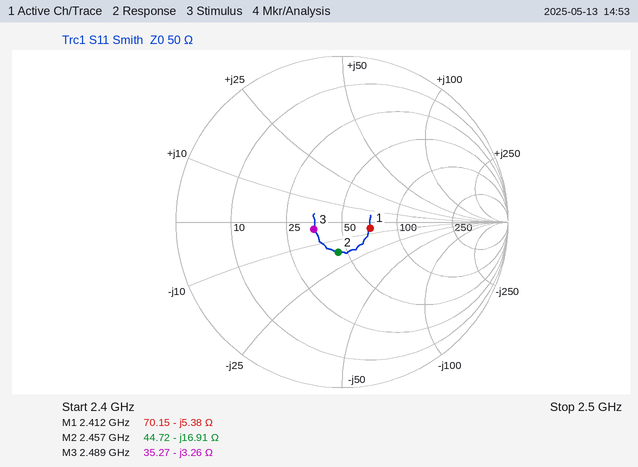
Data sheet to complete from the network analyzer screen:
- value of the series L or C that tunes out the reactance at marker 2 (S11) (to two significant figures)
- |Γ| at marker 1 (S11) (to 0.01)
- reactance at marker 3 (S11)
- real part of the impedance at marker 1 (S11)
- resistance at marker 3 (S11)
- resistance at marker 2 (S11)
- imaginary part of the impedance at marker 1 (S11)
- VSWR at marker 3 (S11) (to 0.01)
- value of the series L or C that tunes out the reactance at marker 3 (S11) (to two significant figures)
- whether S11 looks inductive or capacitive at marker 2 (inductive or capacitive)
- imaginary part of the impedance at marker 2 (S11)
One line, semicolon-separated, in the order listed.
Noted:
1.1 nH; 0.17; -3.26 Ω; 70.15 Ω; 35.27 Ω; 44.72 Ω; -5.38 Ω; 1.43; 210 pH; capacitive; -16.91 Ω
